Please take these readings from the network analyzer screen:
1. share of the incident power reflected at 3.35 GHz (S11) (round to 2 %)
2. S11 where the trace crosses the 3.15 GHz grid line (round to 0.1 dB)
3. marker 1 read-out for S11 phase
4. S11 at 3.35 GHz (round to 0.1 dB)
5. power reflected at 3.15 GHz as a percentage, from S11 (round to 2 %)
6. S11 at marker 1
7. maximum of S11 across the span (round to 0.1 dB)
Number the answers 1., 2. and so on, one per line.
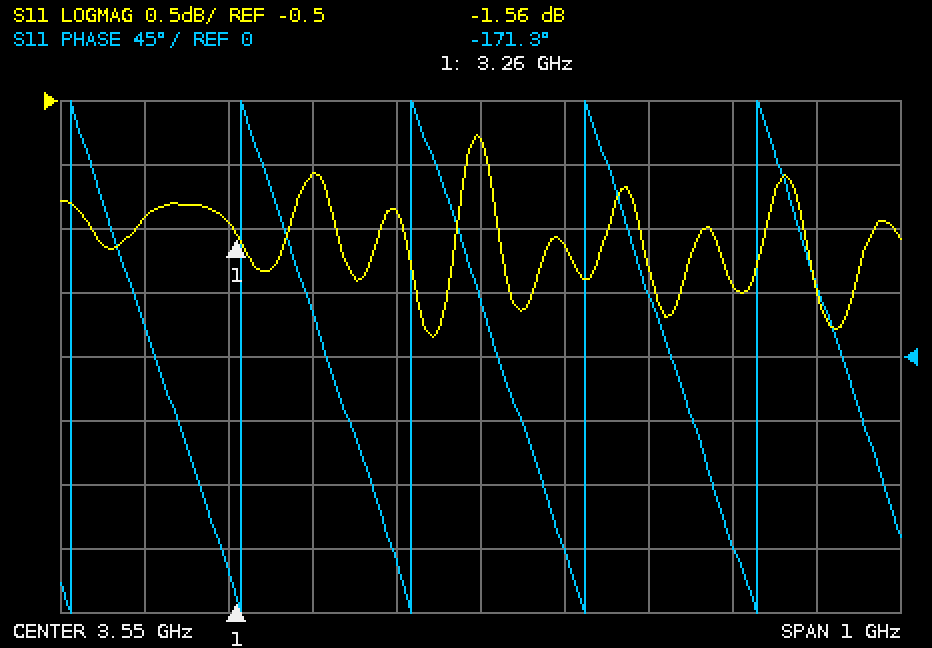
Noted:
1. 78 %
2. -1.4 dB
3. -171.3°
4. -1.1 dB
5. 72 %
6. -1.56 dB
7. -0.8 dB
